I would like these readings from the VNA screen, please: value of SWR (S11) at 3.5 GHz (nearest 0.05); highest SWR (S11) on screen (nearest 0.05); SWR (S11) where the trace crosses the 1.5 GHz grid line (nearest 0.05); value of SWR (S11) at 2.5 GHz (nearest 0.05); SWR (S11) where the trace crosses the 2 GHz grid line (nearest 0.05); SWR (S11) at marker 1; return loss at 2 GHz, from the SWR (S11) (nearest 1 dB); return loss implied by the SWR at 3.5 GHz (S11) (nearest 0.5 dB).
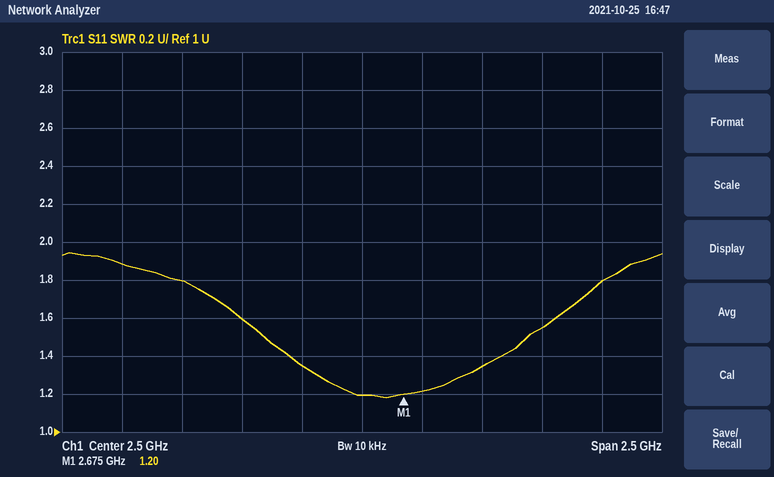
1.80
1.95
1.90
1.20
1.60
1.20
13 dB
11.0 dB
